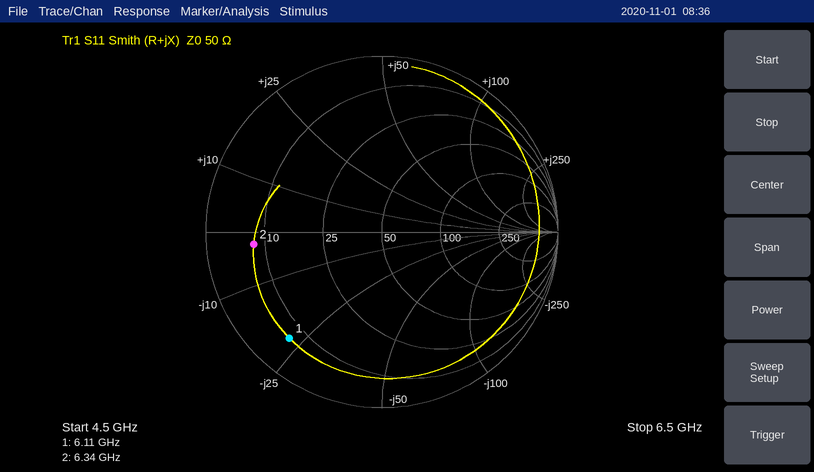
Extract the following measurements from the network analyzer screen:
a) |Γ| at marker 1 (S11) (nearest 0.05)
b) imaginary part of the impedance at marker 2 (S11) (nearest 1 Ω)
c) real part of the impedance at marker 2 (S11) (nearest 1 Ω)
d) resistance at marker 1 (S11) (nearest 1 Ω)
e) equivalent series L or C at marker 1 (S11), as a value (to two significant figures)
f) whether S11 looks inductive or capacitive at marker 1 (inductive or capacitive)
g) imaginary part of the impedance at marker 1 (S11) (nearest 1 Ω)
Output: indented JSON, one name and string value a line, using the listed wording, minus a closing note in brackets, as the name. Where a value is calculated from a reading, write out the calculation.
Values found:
{
  "|Γ| at marker 1 (S11)": "0.80",
  "imaginary part of the impedance at marker 2 (S11)": "-2 Ω",
  "real part of the impedance at marker 2 (S11)": "8 Ω",
  "resistance at marker 1 (S11)": "7 Ω",
  "equivalent series L or C at marker 1 (S11), as a value": "C = 1/(2π × 6.11 GHz × 22 Ω) ≈ 1.2 pF",
  "whether S11 looks inductive or capacitive at marker 1": "capacitive",
  "imaginary part of the impedance at marker 1 (S11)": "-22 Ω"
}
